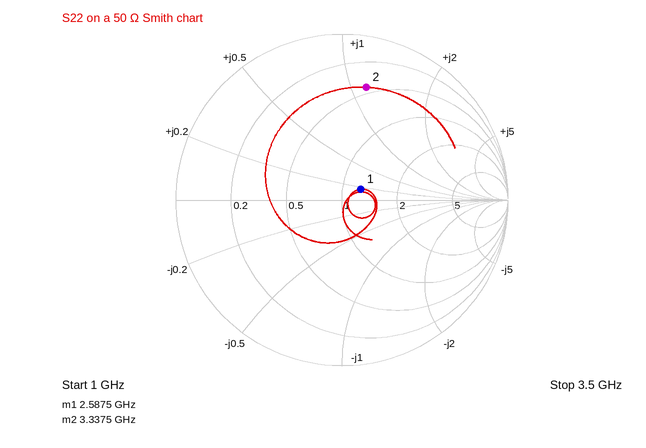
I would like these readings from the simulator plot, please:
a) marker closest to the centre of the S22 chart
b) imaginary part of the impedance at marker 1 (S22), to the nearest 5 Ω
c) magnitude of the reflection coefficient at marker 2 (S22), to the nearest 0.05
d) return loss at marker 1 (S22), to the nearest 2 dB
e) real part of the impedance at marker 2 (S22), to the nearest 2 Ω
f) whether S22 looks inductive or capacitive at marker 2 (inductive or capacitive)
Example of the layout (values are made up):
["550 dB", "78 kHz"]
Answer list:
["marker 1", "+10 Ω", "0.70", "18 dB", "22 Ω", "inductive"]
